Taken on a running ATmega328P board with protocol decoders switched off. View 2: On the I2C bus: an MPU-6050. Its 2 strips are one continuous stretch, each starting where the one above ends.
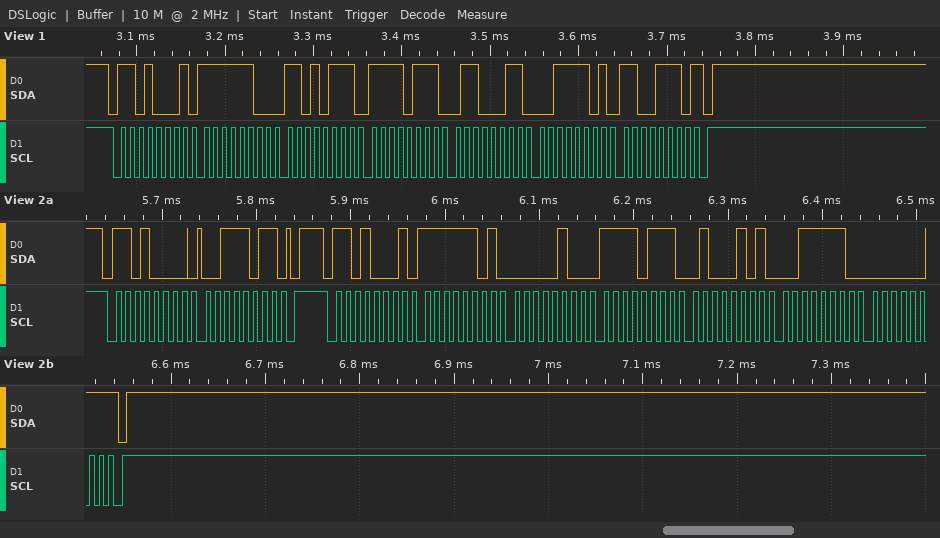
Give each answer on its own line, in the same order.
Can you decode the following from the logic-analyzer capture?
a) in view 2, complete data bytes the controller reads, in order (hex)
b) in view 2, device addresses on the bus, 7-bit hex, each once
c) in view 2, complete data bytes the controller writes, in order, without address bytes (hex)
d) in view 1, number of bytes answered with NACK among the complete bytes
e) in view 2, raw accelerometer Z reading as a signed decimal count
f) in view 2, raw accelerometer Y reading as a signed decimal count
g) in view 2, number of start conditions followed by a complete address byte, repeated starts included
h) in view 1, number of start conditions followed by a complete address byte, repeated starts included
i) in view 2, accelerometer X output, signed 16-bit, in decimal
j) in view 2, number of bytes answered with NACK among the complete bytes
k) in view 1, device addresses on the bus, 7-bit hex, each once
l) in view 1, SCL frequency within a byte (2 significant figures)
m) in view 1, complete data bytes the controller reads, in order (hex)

FD 04 F7 45 3E 03
0x68
3B
1
15875
-2235
2
1
-764
1
0x68
100 kHz
FC D7 F7 63 3D CE
